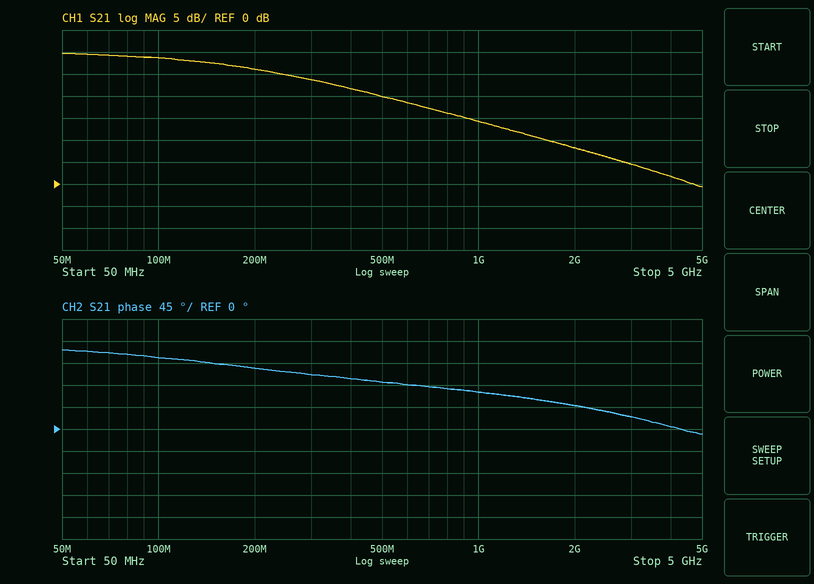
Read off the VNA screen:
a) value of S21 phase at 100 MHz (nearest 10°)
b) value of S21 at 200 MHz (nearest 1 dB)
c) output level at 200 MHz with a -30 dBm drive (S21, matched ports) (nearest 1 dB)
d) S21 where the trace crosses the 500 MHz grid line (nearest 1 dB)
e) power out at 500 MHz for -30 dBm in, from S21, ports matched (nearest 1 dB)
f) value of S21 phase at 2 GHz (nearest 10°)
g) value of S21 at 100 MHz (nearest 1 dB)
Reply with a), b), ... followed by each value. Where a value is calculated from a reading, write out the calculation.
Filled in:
a) 150°
b) 26 dB
c) -30 dBm + (26 dB) = -4 dBm
d) 20 dB
e) -30 dBm + (20 dB) = -10 dBm
f) 50°
g) 29 dB
